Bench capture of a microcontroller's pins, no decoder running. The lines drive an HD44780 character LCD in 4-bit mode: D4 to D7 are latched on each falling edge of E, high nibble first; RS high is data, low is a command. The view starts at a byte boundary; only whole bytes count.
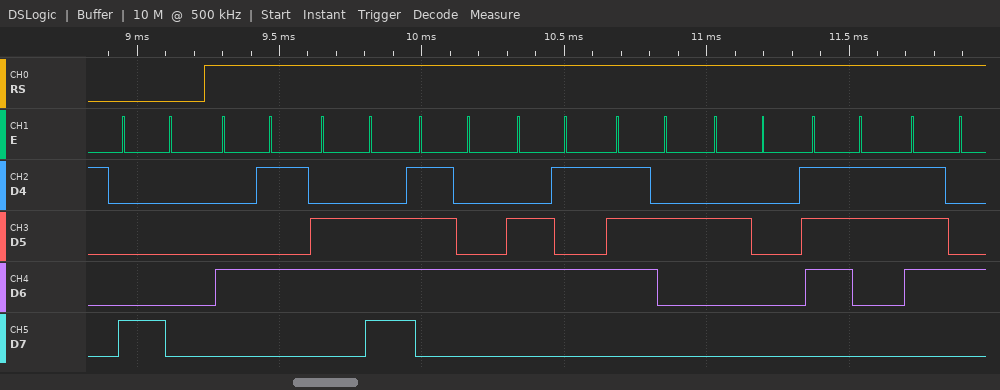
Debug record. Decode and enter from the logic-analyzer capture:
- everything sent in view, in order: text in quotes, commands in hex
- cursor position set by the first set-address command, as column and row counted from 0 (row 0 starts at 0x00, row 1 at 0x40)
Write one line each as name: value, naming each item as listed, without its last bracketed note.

everything sent in view, in order: text in quotes, commands in hex: 0x80 "Enter st"
cursor position set by the first set-address command, as column and row counted from 0: column 0, row 0
